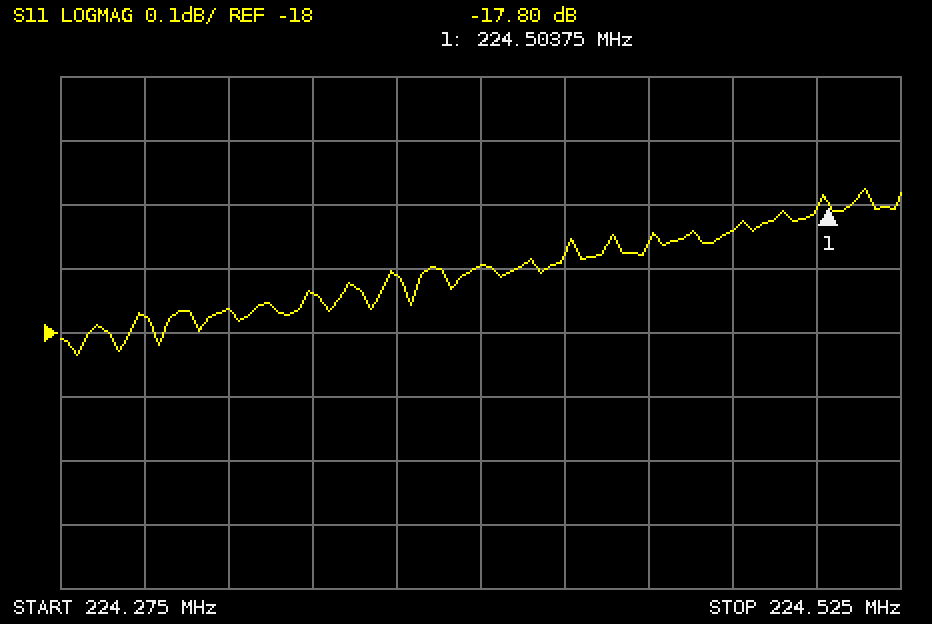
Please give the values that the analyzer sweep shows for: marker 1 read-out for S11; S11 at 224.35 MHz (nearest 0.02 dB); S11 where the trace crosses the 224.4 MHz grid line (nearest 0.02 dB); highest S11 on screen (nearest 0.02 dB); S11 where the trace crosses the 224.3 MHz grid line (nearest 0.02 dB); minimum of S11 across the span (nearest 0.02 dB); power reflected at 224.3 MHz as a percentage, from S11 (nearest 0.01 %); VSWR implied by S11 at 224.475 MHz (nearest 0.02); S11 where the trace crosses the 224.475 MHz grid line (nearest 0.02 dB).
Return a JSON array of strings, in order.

["-17.80 dB", "-17.94 dB", "-17.90 dB", "-17.78 dB", "-17.98 dB", "-18.04 dB", "1.59 %", "1.30", "-17.84 dB"]
